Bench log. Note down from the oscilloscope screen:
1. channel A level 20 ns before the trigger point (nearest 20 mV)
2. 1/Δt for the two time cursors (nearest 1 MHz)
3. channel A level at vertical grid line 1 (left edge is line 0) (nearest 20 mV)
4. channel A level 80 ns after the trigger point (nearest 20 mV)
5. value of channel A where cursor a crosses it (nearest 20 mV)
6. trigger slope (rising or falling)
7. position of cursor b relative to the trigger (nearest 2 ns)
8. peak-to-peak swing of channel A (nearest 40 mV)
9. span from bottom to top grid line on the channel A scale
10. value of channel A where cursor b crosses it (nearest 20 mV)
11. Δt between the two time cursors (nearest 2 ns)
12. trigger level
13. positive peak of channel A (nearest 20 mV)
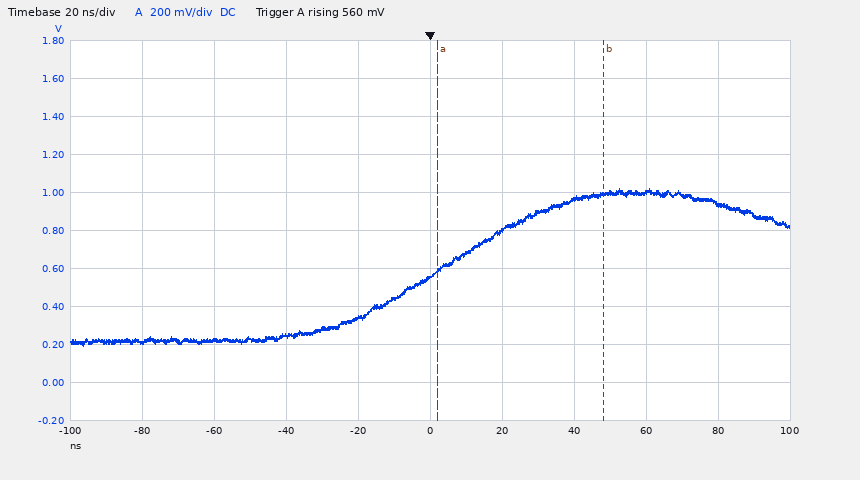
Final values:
340 mV
22 MHz
220 mV
940 mV
580 mV
rising
+48 ns
840 mV
2 V
980 mV
46 ns
560 mV
1.02 V
